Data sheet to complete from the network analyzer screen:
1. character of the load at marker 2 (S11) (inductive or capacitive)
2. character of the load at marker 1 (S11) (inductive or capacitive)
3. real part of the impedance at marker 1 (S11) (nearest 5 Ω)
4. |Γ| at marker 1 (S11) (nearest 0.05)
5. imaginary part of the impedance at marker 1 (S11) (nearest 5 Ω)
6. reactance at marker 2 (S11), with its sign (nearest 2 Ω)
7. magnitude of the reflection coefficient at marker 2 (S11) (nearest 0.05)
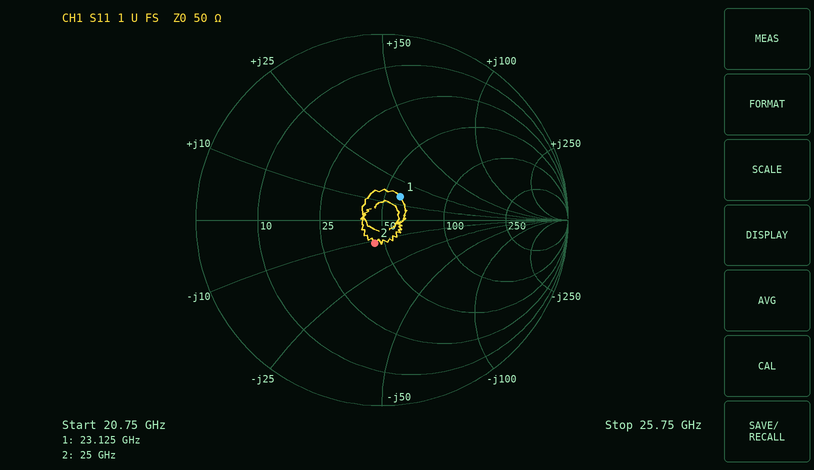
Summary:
capacitive
inductive
60 Ω
0.15
+15 Ω
-12 Ω
0.15
